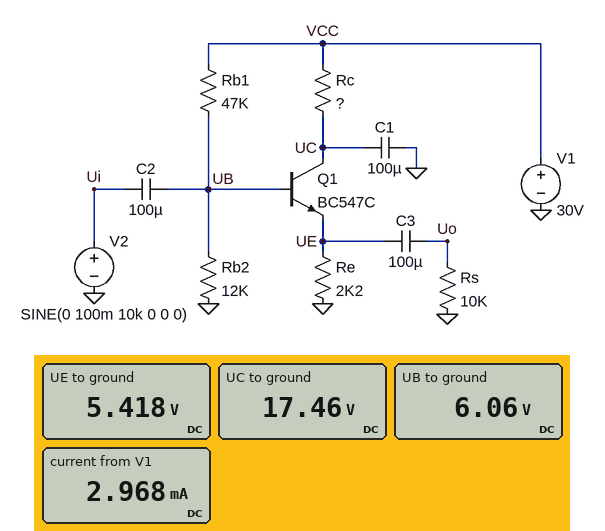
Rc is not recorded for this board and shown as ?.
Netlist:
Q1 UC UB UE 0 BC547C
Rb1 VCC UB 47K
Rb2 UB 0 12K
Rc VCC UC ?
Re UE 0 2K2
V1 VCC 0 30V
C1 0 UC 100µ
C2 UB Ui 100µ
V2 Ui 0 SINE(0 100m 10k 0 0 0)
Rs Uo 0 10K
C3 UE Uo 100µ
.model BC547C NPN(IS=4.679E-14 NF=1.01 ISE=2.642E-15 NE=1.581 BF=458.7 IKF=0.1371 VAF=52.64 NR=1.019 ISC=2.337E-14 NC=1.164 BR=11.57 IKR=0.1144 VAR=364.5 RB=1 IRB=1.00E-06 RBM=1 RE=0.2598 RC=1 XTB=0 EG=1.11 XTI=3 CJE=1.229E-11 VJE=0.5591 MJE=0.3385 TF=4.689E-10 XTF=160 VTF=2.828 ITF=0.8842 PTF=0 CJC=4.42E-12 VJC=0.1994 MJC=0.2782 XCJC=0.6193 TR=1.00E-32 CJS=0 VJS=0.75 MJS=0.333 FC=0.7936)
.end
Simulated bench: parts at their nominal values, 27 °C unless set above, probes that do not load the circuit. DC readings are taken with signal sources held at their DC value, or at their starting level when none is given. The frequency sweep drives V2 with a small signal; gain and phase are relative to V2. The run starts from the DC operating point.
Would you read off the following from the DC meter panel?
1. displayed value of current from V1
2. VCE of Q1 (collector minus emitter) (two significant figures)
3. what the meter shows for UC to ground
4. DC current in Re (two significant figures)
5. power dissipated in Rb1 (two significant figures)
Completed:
2.968 mA
12 V
17.46 V
2.5 mA
12 mW
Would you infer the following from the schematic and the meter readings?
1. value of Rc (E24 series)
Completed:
5.1 kΩ
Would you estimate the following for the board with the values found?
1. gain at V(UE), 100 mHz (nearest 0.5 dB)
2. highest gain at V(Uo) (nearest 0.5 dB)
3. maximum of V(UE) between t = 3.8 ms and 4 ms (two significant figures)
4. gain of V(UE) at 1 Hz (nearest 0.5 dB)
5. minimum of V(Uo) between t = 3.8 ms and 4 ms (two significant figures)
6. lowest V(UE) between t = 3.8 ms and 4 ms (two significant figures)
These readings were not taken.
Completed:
-6.0 dB
0 dB
5.5 V
0 dB
-99 mV
5.3 V
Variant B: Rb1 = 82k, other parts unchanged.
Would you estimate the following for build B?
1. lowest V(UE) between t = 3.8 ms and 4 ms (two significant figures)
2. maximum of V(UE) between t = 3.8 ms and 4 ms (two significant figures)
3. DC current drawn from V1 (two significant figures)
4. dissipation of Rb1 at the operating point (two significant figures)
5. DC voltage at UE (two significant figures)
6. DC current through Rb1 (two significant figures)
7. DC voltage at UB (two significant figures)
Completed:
3.1 V
3.3 V
1.8 mA
8.4 mW
3.2 V
320 µA
3.8 V
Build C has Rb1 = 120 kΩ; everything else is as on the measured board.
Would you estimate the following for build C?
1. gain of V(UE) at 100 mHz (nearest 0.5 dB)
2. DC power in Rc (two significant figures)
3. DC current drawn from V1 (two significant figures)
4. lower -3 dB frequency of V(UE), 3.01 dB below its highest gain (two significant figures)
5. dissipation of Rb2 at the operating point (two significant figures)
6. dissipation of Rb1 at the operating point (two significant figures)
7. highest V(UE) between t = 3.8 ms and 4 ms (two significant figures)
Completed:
-5.0 dB
4.6 mW
1.2 mA
150 mHz
610 µW
6.2 mW
2.2 V
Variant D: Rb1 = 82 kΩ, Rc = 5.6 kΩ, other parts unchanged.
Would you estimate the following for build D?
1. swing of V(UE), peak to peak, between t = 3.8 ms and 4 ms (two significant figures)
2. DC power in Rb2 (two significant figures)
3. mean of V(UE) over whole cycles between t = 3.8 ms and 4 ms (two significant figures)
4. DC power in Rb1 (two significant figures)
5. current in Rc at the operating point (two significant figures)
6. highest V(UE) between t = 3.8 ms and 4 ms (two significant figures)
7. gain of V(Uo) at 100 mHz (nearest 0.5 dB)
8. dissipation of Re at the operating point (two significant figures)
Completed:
200 mV
1.2 mW
3.2 V
8.4 mW
1.4 mA
3.3 V
-11.0 dB
4.6 mW
